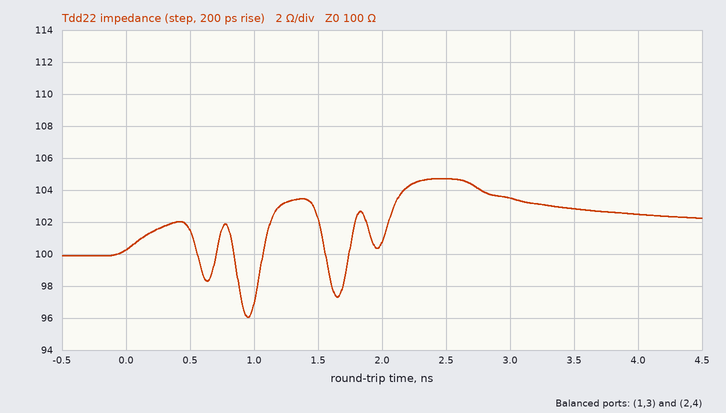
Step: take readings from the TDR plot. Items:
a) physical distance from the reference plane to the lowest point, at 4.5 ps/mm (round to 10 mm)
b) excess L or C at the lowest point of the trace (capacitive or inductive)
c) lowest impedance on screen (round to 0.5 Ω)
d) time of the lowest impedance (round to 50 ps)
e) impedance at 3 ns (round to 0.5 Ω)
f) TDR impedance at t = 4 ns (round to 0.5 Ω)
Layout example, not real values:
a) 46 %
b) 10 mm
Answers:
a) 110 mm
b) capacitive
c) 96.0 Ω
d) 950 ps
e) 103.5 Ω
f) 102.5 Ω
